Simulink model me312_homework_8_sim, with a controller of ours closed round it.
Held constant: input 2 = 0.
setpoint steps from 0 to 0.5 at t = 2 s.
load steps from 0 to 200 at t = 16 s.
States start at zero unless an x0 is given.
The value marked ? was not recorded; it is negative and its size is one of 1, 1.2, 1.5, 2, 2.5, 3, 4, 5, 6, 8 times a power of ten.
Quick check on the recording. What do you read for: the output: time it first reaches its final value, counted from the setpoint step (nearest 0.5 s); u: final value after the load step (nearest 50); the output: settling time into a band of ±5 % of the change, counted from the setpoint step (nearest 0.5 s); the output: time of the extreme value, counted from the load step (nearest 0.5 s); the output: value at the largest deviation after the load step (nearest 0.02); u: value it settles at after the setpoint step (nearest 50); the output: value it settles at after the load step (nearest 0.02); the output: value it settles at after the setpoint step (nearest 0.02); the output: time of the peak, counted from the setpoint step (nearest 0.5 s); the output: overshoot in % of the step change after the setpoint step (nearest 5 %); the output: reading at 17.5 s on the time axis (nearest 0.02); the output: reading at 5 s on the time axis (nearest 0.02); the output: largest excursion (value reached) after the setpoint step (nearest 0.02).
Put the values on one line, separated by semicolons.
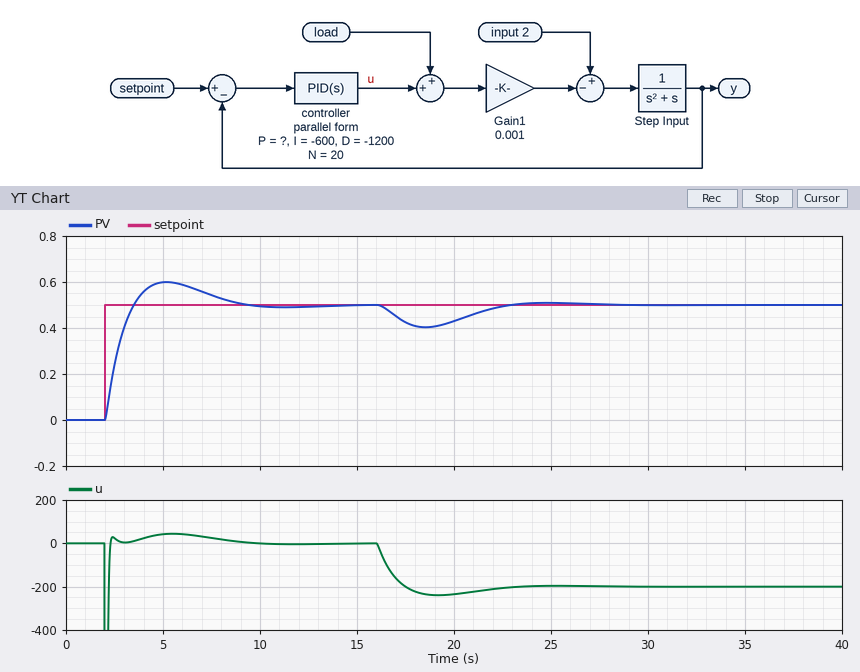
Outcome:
1.5 s; -200; 6.0 s; 2.5 s; 0.40; 0; 0.50; 0.50; 3.0 s; 20 %; 0.42; 0.60; 0.60
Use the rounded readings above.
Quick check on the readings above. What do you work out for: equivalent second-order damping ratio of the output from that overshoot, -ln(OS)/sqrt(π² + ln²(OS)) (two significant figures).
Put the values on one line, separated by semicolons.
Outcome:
0.46
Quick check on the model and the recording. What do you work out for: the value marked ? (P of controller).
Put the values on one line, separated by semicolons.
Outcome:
-1500
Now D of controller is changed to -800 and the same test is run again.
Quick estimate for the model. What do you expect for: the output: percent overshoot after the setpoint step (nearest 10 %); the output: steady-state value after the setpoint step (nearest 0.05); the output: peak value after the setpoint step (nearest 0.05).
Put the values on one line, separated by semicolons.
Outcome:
30 %; 0.50; 0.65
